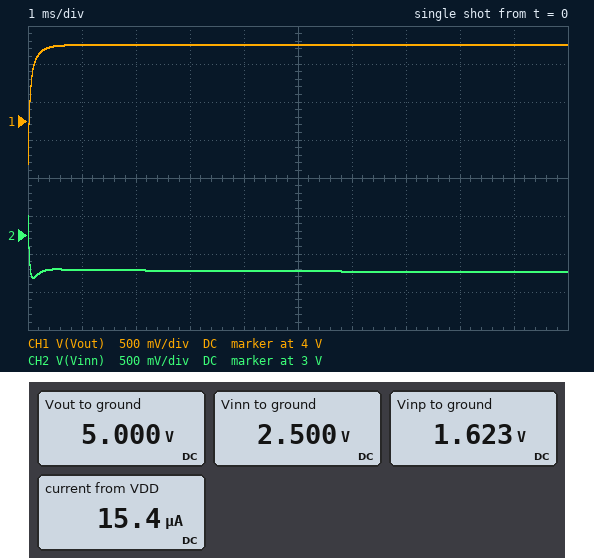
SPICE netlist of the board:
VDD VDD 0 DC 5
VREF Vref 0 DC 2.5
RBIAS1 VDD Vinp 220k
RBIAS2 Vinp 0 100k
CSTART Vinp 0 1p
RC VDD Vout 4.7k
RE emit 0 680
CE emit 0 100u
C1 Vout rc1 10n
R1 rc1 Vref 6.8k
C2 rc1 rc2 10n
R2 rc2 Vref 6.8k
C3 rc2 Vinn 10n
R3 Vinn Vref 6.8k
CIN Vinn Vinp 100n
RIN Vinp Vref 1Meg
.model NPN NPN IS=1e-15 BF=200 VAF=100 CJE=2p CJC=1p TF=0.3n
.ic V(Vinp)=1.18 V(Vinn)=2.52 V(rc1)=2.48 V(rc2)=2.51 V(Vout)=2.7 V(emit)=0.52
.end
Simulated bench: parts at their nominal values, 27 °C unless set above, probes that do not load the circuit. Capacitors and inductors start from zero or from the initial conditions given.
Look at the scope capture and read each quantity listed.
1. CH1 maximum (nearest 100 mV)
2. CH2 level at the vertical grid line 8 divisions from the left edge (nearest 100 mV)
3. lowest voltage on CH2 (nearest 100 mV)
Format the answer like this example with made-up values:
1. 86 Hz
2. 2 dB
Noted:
1. 5.0 V
2. 2.5 V
3. 2.4 V
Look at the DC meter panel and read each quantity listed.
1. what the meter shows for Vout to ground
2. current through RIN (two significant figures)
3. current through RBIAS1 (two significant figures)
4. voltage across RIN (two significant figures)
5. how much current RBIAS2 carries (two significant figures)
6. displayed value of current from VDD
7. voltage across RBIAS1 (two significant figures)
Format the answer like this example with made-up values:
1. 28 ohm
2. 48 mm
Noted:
1. 5.000 V
2. 880 nA
3. 15 µA
4. 880 mV
5. 16 µA
6. 15.4 µA
7. 3.4 V
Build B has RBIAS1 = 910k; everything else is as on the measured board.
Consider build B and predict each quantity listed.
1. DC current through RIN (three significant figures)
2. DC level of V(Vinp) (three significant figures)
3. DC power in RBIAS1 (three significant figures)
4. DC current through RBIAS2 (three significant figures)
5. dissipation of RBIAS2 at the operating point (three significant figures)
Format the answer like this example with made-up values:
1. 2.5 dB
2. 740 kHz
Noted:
1. 1.84 µA
2. 661 mV
3. 20.7 µW
4. 6.61 µA
5. 4.37 µW
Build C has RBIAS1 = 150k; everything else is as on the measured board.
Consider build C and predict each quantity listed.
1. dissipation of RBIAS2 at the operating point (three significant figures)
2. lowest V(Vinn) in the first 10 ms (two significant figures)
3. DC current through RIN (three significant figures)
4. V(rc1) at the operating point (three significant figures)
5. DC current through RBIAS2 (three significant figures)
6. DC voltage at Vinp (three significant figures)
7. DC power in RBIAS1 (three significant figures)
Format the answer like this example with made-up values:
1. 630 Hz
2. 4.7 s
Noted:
1. 41.1 µW
2. 2.5 V
3. 472 nA
4. 2.50 V
5. 20.3 µA
6. 2.03 V
7. 58.9 µW
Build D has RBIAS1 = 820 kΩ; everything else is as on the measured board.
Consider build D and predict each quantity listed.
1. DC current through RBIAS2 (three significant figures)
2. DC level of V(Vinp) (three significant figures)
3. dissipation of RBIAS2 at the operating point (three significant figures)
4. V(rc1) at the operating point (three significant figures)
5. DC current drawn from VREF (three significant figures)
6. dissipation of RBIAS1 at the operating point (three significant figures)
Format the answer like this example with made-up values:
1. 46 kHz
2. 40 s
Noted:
1. 7.04 µA
2. 704 mV
3. 4.95 µW
4. 2.50 V
5. 1.80 µA
6. 22.5 µW
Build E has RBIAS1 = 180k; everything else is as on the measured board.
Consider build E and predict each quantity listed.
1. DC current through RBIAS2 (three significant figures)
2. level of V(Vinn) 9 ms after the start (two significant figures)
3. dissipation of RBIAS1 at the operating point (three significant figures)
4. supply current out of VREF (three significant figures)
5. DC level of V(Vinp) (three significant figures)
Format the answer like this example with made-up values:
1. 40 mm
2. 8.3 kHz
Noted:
1. 18.3 µA
2. 2.5 V
3. 55.9 µW
4. 671 nA
5. 1.83 V
